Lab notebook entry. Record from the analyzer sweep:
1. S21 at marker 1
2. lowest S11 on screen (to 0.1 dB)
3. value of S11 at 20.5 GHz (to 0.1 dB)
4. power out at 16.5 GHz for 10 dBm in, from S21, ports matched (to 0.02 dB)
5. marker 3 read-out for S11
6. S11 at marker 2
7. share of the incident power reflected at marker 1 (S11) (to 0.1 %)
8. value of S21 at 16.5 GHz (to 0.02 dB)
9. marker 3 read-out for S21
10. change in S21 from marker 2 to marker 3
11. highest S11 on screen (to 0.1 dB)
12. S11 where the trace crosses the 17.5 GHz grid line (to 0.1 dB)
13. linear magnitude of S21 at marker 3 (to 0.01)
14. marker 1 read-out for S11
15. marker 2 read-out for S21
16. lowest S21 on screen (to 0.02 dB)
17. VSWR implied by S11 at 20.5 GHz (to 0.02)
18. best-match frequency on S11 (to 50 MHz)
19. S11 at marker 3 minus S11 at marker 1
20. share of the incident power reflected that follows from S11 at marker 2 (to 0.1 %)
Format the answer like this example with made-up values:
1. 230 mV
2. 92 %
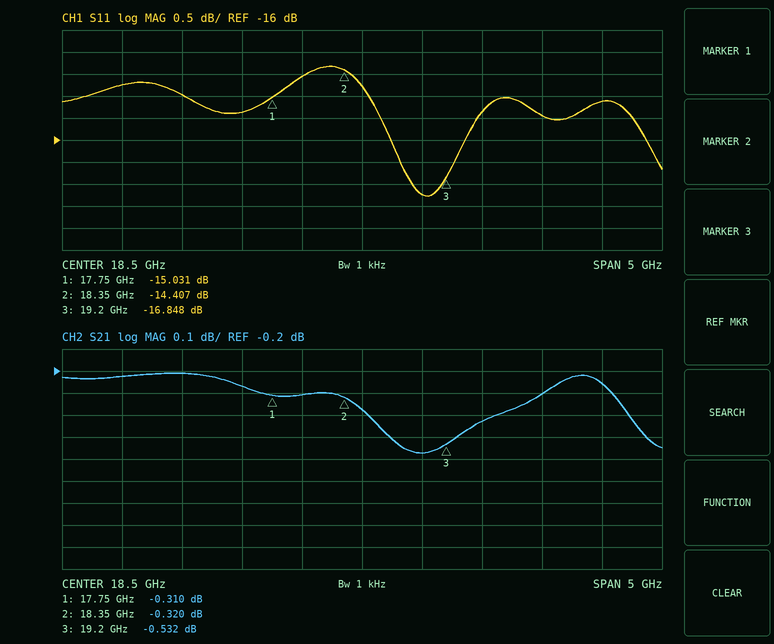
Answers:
1. -0.310 dB
2. -17.3 dB
3. -15.1 dB
4. 9.78 dBm
5. -16.848 dB
6. -14.407 dB
7. 3.1 %
8. -0.22 dB
9. -0.532 dB
10. -0.212 dB
11. -14.3 dB
12. -15.4 dB
13. 0.94
14. -15.031 dB
15. -0.320 dB
16. -0.58 dB
17. 1.42
18. 19.05 GHz
19. -1.817 dB
20. 3.6 %
